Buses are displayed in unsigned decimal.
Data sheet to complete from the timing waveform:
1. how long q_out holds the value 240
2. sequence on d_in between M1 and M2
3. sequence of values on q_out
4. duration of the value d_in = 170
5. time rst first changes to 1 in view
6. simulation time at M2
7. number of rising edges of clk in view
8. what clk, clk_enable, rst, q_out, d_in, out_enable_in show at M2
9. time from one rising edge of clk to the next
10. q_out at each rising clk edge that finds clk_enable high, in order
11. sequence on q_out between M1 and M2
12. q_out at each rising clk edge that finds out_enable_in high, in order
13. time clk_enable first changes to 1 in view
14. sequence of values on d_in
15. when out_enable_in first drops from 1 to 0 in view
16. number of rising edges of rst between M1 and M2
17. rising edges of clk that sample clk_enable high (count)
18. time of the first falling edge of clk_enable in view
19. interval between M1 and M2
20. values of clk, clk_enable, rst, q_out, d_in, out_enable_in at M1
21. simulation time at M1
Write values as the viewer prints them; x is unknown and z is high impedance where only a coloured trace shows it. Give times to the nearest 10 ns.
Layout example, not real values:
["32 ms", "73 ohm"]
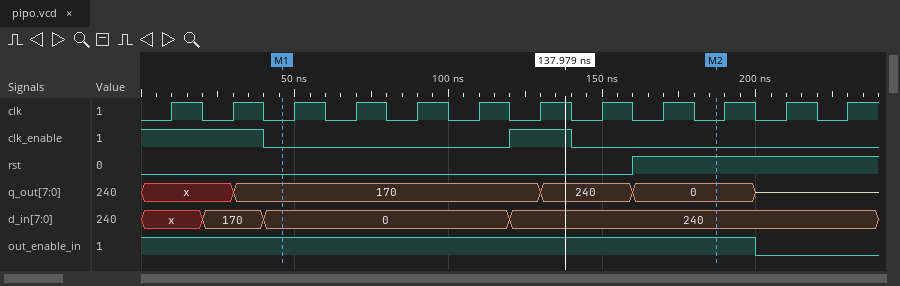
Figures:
["30 ns", "0, 240", "x, 170, 240, 0, z", "20 ns", "160 ns", "190 ns", "12", "clk=0, clk_enable=0, rst=1, q_out=0, d_in=240, out_enable_in=1", "20 ns", "x, x, 170", "170, 240, 0", "x, x, 170, 170, 170, 170, 170, 240, 0, 0", "120 ns", "x, 170, 0, 240", "200 ns", "1", "3", "40 ns", "140 ns", "clk=0, clk_enable=0, rst=0, q_out=170, d_in=0, out_enable_in=1", "50 ns"]
